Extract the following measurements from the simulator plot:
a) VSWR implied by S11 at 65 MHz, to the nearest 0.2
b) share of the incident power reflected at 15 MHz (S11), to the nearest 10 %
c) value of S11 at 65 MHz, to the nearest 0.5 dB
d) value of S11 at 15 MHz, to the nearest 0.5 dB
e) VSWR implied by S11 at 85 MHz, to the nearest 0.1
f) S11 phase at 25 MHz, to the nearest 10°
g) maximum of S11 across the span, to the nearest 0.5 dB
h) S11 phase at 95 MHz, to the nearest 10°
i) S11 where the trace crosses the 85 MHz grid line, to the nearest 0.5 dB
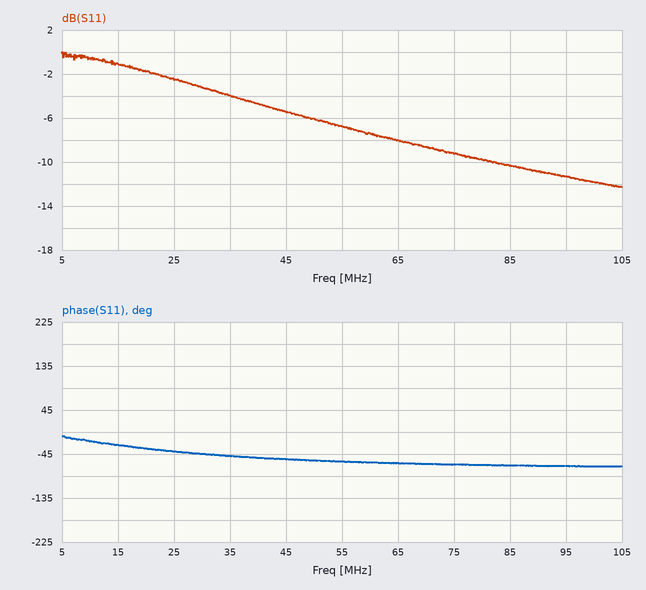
2.4
80 %
-8.0 dB
-1.0 dB
1.9
-40°
0.0 dB
-70°
-10.5 dB
